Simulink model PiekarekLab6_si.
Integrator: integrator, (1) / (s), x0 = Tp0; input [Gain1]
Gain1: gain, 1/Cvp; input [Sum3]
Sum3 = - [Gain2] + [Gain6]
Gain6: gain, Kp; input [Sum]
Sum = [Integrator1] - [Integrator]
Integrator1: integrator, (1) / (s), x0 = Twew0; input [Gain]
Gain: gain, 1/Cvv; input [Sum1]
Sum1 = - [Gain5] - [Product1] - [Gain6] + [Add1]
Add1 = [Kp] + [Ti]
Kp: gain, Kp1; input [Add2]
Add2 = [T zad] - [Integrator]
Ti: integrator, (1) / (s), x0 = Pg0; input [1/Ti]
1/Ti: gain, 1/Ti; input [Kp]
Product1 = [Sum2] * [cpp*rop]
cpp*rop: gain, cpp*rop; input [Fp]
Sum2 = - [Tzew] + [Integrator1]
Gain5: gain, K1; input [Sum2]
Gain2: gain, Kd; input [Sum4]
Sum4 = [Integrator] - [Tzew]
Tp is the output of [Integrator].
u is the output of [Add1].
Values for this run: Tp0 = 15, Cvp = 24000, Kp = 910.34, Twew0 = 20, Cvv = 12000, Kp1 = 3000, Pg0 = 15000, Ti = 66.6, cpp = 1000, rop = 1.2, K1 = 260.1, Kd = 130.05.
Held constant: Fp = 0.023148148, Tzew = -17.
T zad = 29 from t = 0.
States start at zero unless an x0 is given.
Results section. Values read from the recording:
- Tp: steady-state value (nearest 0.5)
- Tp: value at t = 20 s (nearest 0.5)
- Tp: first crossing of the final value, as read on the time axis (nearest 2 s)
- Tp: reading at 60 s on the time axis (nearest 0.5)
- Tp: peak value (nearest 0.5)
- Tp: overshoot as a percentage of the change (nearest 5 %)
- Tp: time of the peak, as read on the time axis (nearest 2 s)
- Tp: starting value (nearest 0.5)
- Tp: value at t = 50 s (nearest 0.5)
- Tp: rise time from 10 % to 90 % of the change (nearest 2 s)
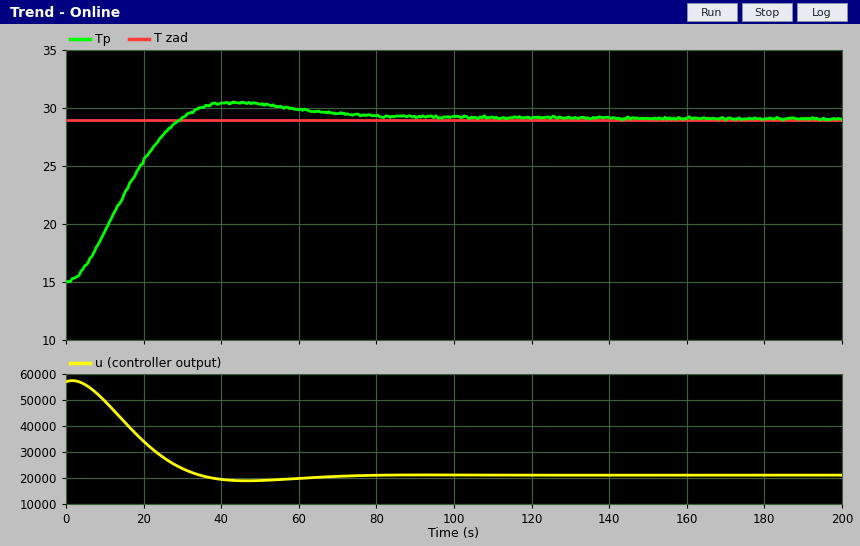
29.0
25.5
30 s
30.0
30.5
10 %
44 s
15.0
30.5
20 s
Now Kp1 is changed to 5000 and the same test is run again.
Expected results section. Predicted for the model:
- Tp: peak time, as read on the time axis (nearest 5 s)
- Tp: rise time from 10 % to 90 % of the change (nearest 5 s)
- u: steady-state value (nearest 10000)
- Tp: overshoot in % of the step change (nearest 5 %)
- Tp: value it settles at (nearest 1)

30 s
15 s
20000
20 %
29
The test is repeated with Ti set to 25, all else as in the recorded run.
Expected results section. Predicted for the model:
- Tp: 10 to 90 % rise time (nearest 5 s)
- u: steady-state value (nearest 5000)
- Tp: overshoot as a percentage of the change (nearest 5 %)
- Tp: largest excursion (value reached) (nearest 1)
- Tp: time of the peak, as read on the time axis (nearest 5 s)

15 s
20000
35 %
34
40 s
